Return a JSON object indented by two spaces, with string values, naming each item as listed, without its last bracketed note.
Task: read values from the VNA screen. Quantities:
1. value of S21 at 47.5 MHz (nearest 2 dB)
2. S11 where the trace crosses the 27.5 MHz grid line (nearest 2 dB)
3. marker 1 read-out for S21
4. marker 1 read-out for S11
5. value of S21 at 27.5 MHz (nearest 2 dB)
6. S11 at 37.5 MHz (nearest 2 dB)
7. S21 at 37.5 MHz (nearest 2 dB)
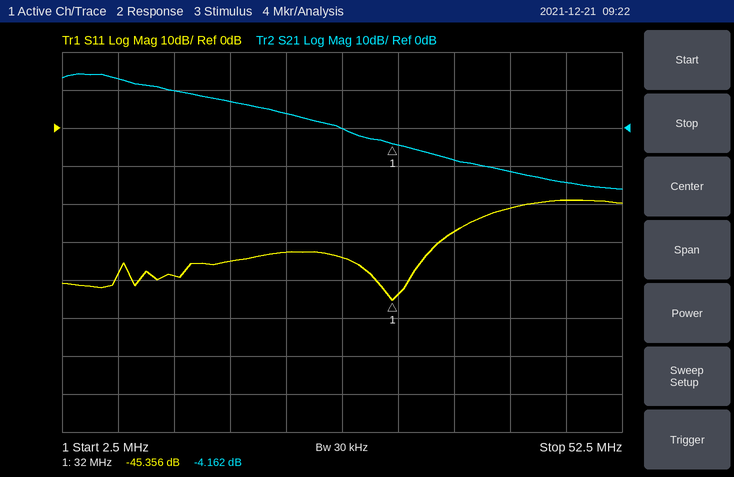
{
  "value of S21 at 47.5 MHz": "-14 dB",
  "S11 where the trace crosses the 27.5 MHz grid line": "-34 dB",
  "marker 1 read-out for S21": "-4.162 dB",
  "marker 1 read-out for S11": "-45.356 dB",
  "value of S21 at 27.5 MHz": "0 dB",
  "S11 at 37.5 MHz": "-28 dB",
  "S21 at 37.5 MHz": "-8 dB"
}
